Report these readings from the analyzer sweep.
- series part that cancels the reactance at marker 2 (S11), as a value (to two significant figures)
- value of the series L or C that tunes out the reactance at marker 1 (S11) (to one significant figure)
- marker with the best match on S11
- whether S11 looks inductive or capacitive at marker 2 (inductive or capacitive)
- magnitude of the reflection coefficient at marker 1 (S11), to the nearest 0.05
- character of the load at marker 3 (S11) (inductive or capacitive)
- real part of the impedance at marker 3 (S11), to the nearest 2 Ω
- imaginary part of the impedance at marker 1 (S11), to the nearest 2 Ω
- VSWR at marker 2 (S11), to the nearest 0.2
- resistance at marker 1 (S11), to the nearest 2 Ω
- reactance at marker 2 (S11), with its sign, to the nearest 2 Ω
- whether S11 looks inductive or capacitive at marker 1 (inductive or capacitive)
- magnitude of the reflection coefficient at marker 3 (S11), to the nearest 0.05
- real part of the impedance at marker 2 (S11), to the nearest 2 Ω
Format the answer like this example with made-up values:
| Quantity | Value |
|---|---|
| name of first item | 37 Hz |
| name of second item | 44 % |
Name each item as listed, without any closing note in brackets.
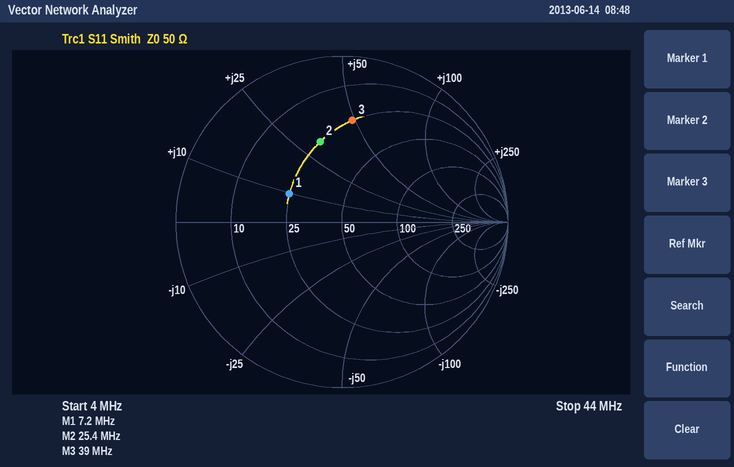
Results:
| Quantity | Value |
|---|---|
| series part that cancels the reactance at marker 2 (S11), as a value | 200 pF |
| value of the series L or C that tunes out the reactance at marker 1 (S11) | 2 nF |
| marker with the best match on S11 | marker 1 |
| whether S11 looks inductive or capacitive at marker 2 | inductive |
| magnitude of the reflection coefficient at marker 1 (S11), to the nearest 0.05 | 0.35 |
| character of the load at marker 3 (S11) | inductive |
| real part of the impedance at marker 3 (S11), to the nearest 2 Ω | 24 Ω |
| imaginary part of the impedance at marker 1 (S11), to the nearest 2 Ω | +10 Ω |
| VSWR at marker 2 (S11), to the nearest 0.2 | 3.0 |
| resistance at marker 1 (S11), to the nearest 2 Ω | 24 Ω |
| reactance at marker 2 (S11), with its sign, to the nearest 2 Ω | +32 Ω |
| whether S11 looks inductive or capacitive at marker 1 | inductive |
| magnitude of the reflection coefficient at marker 3 (S11), to the nearest 0.05 | 0.60 |
| real part of the impedance at marker 2 (S11), to the nearest 2 Ω | 24 Ω |
